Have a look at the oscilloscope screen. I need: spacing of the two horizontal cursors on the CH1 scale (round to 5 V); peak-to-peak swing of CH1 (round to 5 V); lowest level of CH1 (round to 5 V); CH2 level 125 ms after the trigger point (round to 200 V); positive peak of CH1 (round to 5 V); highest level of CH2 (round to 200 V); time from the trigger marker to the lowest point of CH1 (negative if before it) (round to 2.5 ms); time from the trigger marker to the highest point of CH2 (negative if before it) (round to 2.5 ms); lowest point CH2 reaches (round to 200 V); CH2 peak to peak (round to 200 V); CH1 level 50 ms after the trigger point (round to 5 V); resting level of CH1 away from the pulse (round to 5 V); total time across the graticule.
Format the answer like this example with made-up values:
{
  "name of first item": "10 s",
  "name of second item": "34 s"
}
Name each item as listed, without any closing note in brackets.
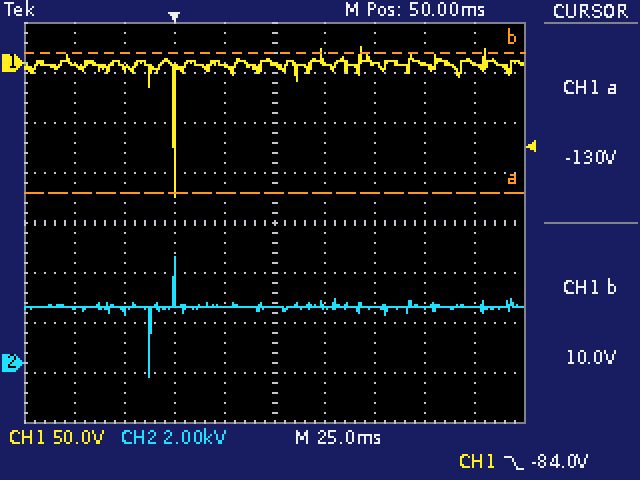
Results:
{
  "spacing of the two horizontal cursors on the CH1 scale": "140 V",
  "peak-to-peak swing of CH1": "150 V",
  "lowest level of CH1": "-135 V",
  "CH2 level 125 ms after the trigger point": "2.2 kV",
  "positive peak of CH1": "15 V",
  "highest level of CH2": "4.2 kV",
  "time from the trigger marker to the lowest point of CH1 (negative if before it)": "0.0 ms",
  "time from the trigger marker to the highest point of CH2 (negative if before it)": "0.0 ms",
  "lowest point CH2 reaches": "-600 V",
  "CH2 peak to peak": "4.8 kV",
  "CH1 level 50 ms after the trigger point": "0 V",
  "resting level of CH1 away from the pulse": "0 V",
  "total time across the graticule": "250 ms"
}
